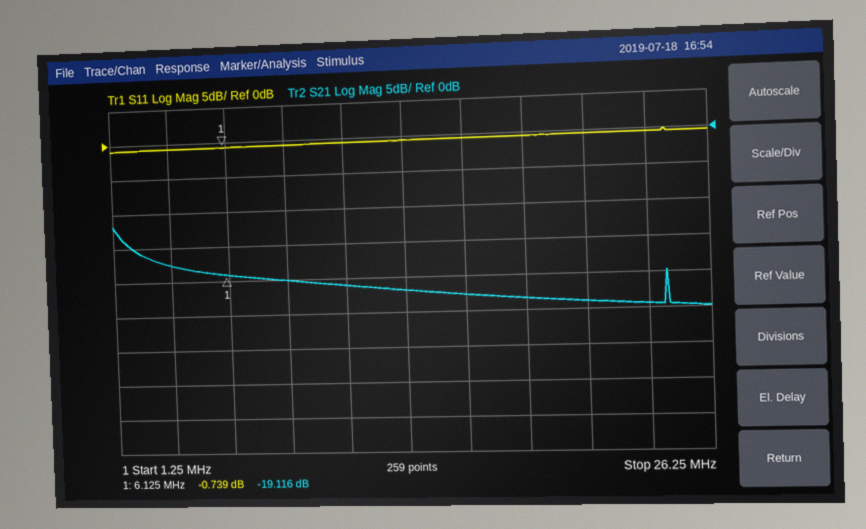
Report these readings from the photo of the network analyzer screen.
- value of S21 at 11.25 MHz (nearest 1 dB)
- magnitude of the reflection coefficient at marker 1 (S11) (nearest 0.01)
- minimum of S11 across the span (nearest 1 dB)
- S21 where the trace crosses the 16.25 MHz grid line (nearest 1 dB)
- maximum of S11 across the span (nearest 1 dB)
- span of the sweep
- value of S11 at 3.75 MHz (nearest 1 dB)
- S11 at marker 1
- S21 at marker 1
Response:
-21 dB
0.92
-1 dB
-23 dB
0 dB
25 MHz
-1 dB
-0.739 dB
-19.116 dB
